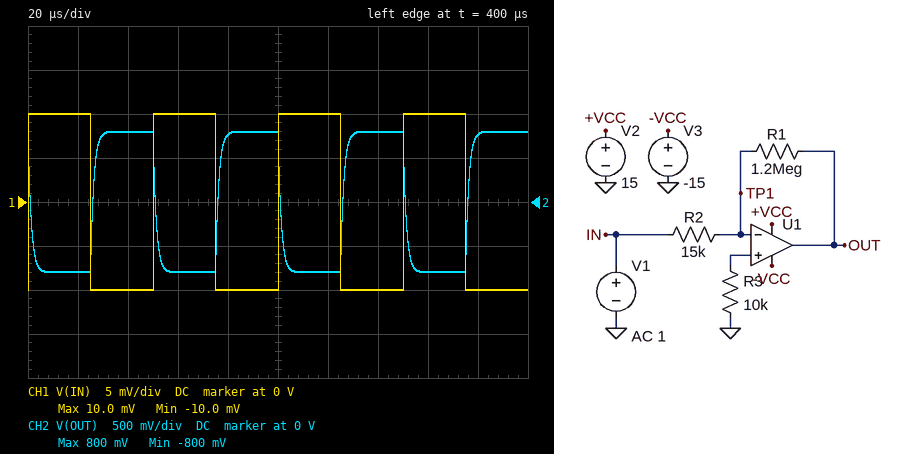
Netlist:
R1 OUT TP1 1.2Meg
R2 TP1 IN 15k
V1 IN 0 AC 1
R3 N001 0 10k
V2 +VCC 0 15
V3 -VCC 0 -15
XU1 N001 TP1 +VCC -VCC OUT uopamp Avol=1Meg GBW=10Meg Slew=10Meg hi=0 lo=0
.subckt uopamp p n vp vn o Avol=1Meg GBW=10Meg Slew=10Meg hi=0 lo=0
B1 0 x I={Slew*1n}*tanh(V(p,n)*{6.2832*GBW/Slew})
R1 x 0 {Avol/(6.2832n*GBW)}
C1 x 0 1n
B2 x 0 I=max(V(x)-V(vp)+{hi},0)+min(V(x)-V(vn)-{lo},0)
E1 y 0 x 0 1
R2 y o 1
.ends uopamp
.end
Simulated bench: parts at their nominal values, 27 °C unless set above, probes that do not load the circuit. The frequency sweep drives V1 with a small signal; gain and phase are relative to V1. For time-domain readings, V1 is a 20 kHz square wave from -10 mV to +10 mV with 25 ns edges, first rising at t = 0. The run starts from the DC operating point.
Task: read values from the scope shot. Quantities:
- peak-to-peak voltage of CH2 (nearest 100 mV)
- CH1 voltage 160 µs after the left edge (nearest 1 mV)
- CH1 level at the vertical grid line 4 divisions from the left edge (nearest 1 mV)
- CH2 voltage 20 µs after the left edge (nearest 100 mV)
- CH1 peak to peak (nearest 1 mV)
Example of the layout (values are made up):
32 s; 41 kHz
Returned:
1.6 V; 10 mV; -10 mV; -800 mV; 20 mV
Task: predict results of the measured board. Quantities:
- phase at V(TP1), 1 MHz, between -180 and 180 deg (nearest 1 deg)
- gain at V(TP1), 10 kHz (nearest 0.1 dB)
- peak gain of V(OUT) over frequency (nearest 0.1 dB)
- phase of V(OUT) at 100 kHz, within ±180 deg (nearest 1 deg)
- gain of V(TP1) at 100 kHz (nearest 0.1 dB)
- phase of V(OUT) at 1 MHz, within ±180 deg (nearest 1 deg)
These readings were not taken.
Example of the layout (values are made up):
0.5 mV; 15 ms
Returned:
7 deg; -22.0 dB; 38.1 dB; 141 deg; -4.1 dB; 97 deg
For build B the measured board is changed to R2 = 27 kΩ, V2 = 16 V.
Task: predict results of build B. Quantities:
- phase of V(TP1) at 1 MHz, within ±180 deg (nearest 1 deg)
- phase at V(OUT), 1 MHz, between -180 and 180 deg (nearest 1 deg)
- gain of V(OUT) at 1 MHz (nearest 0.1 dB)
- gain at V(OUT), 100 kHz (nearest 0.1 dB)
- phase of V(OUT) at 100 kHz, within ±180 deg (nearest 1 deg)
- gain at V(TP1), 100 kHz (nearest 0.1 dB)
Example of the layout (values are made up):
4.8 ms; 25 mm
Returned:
12 deg; 102 deg; 19.6 dB; 32.1 dB; 156 deg; -7.9 dB
